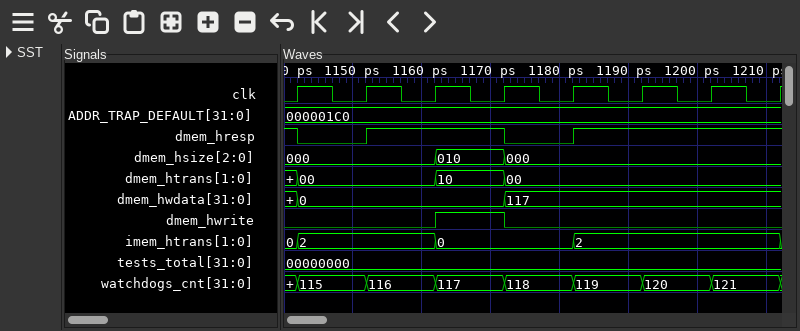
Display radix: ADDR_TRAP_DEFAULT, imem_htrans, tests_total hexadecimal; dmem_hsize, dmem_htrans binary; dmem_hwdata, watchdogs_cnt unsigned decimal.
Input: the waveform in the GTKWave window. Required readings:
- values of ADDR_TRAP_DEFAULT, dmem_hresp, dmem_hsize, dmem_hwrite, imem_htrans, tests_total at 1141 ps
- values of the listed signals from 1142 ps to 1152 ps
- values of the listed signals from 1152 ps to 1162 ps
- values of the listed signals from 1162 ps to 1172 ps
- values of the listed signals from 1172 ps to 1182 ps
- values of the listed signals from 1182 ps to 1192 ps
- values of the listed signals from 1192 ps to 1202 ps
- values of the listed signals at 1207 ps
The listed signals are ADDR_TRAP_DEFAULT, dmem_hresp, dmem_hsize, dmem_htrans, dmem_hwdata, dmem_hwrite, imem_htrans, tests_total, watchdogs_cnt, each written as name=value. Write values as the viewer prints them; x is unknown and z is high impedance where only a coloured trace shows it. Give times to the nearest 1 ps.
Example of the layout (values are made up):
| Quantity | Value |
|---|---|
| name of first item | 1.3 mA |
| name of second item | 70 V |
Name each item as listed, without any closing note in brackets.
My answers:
| Quantity | Value |
|---|---|
| values of ADDR_TRAP_DEFAULT, dmem_hresp, dmem_hsize, dmem_hwrite, imem_htrans, tests_total at 1141 ps | ADDR_TRAP_DEFAULT=000001C0, dmem_hresp=1, dmem_hsize=000, dmem_hwrite=0, imem_htrans=0, tests_total=00000000 |
| values of the listed signals from 1142 ps to 1152 ps | ADDR_TRAP_DEFAULT=000001C0, dmem_hresp=0, dmem_hsize=000, dmem_htrans=00, dmem_hwdata=0, dmem_hwrite=0, imem_htrans=2, tests_total=00000000, watchdogs_cnt=115 |
| values of the listed signals from 1152 ps to 1162 ps | ADDR_TRAP_DEFAULT=000001C0, dmem_hresp=1, dmem_hsize=000, dmem_htrans=00, dmem_hwdata=0, dmem_hwrite=0, imem_htrans=2, tests_total=00000000, watchdogs_cnt=116 |
| values of the listed signals from 1162 ps to 1172 ps | ADDR_TRAP_DEFAULT=000001C0, dmem_hresp=1, dmem_hsize=010, dmem_htrans=10, dmem_hwdata=0, dmem_hwrite=1, imem_htrans=0, tests_total=00000000, watchdogs_cnt=117 |
| values of the listed signals from 1172 ps to 1182 ps | ADDR_TRAP_DEFAULT=000001C0, dmem_hresp=0, dmem_hsize=000, dmem_htrans=00, dmem_hwdata=117, dmem_hwrite=0, imem_htrans=0, tests_total=00000000, watchdogs_cnt=118 |
| values of the listed signals from 1182 ps to 1192 ps | ADDR_TRAP_DEFAULT=000001C0, dmem_hresp=1, dmem_hsize=000, dmem_htrans=00, dmem_hwdata=117, dmem_hwrite=0, imem_htrans=2, tests_total=00000000, watchdogs_cnt=119 |
| values of the listed signals from 1192 ps to 1202 ps | ADDR_TRAP_DEFAULT=000001C0, dmem_hresp=1, dmem_hsize=000, dmem_htrans=00, dmem_hwdata=117, dmem_hwrite=0, imem_htrans=2, tests_total=00000000, watchdogs_cnt=120 |
| values of the listed signals at 1207 ps | ADDR_TRAP_DEFAULT=000001C0, dmem_hresp=1, dmem_hsize=000, dmem_htrans=00, dmem_hwdata=117, dmem_hwrite=0, imem_htrans=2, tests_total=00000000, watchdogs_cnt=121 |
